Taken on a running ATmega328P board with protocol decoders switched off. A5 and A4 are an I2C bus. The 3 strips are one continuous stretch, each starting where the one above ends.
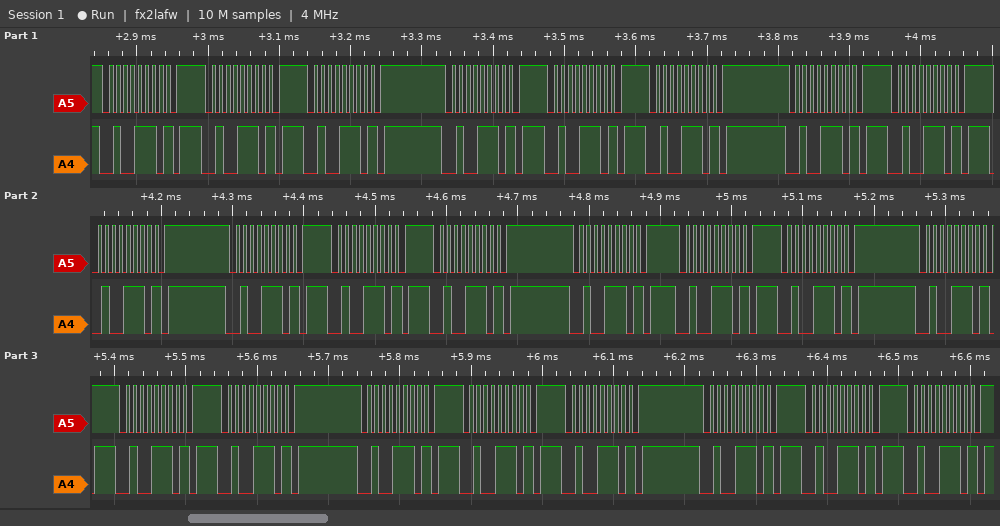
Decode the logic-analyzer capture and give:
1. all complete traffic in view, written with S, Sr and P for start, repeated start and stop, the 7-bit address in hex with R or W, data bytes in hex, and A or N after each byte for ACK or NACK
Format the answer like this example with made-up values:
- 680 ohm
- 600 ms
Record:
- S 27W N P S 27W N P S 27W N P S 27W N P S 27W N P S 27W N P S 27W N P S 27W N P S 27W N P S 27W N P S 27W N P S 27W N P S 27W N P S 27W N P S 27W N P S 27W N P S 27W N P S 27W N P S 27W N P S 27W N P S 27W N P S 27W N P S 27W N P S 27W N P
